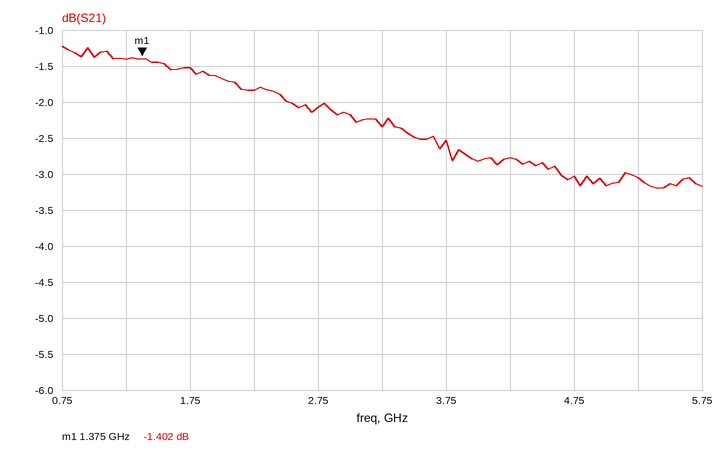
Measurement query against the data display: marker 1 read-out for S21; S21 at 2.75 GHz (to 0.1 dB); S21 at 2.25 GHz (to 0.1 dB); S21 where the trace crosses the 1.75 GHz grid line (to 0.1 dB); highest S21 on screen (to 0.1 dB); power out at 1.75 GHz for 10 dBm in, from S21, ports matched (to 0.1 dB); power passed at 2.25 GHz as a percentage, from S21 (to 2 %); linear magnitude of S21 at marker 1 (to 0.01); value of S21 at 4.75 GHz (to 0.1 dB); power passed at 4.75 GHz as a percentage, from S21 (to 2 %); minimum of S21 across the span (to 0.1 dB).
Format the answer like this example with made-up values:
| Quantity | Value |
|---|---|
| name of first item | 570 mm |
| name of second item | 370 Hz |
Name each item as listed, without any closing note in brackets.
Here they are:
| Quantity | Value |
|---|---|
| marker 1 read-out for S21 | -1.402 dB |
| S21 at 2.75 GHz | -2.1 dB |
| S21 at 2.25 GHz | -1.8 dB |
| S21 where the trace crosses the 1.75 GHz grid line | -1.5 dB |
| highest S21 on screen | -1.2 dB |
| power out at 1.75 GHz for 10 dBm in, from S21, ports matched | 8.5 dBm |
| power passed at 2.25 GHz as a percentage, from S21 | 66 % |
| linear magnitude of S21 at marker 1 | 0.85 |
| value of S21 at 4.75 GHz | -3.0 dB |
| power passed at 4.75 GHz as a percentage, from S21 | 50 % |
| minimum of S21 across the span | -3.2 dB |
